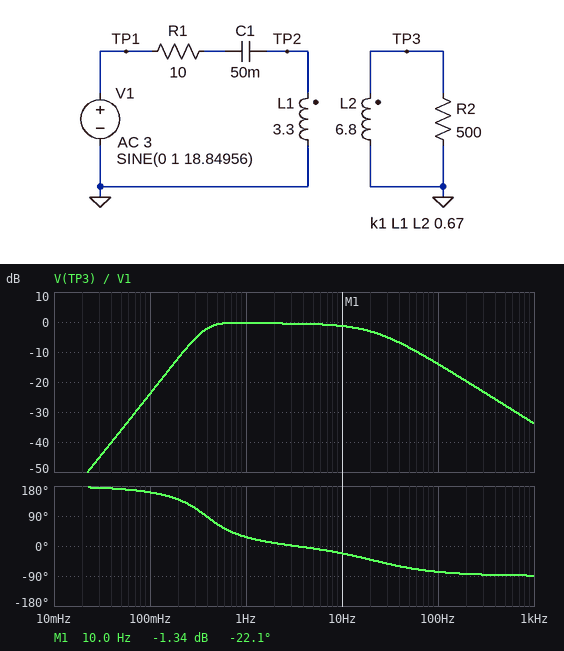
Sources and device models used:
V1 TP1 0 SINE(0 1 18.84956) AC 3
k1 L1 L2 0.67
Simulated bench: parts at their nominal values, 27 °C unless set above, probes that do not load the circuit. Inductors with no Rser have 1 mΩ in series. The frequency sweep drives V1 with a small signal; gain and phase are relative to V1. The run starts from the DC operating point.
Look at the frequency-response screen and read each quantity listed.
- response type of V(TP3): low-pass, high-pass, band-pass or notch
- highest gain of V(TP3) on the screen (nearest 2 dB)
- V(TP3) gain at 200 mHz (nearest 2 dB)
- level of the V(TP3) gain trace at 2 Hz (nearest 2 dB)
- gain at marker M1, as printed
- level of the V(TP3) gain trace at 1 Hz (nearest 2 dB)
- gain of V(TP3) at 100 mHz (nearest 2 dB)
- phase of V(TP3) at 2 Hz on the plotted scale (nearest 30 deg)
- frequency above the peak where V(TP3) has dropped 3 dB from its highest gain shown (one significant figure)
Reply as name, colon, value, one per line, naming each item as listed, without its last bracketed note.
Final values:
response type of V(TP3): low-pass, high-pass, band-pass or notch: band-pass
highest gain of V(TP3) on the screen: 0 dB
V(TP3) gain at 200 mHz: -12 dB
level of the V(TP3) gain trace at 2 Hz: 0 dB
gain at marker M1, as printed: -1.34 dB
level of the V(TP3) gain trace at 1 Hz: 0 dB
gain of V(TP3) at 100 mHz: -24 dB
phase of V(TP3) at 2 Hz on the plotted scale: 0 deg
frequency above the peak where V(TP3) has dropped 3 dB from its highest gain shown: 20 Hz
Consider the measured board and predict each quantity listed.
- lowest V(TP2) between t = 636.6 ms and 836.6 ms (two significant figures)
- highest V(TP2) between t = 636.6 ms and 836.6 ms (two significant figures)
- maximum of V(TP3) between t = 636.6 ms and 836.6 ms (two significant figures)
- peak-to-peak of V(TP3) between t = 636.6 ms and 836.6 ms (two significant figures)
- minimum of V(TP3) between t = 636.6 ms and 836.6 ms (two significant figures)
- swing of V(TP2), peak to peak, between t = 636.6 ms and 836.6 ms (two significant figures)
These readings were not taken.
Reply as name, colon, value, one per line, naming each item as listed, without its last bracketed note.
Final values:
lowest V(TP2) between t = 636.6 ms and 836.6 ms: -990 mV
highest V(TP2) between t = 636.6 ms and 836.6 ms: 990 mV
maximum of V(TP3) between t = 636.6 ms and 836.6 ms: 710 mV
peak-to-peak of V(TP3) between t = 636.6 ms and 836.6 ms: 1.4 V
minimum of V(TP3) between t = 636.6 ms and 836.6 ms: -720 mV
swing of V(TP2), peak to peak, between t = 636.6 ms and 836.6 ms: 2.0 V
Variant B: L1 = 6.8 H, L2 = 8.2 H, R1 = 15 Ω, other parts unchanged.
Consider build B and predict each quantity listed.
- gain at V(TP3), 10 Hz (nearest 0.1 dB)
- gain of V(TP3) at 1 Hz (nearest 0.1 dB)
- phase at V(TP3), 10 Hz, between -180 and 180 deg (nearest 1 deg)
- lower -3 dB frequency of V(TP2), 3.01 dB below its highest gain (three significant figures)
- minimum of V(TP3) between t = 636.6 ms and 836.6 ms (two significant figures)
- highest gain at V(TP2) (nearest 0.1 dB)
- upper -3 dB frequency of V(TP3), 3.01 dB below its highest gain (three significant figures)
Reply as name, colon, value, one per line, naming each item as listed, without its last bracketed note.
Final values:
gain at V(TP3), 10 Hz: -4.0 dB
gain of V(TP3) at 1 Hz: -2.7 dB
phase at V(TP3), 10 Hz, between -180 and 180 deg: -27 deg
lower -3 dB frequency of V(TP2), 3.01 dB below its highest gain: 252 mHz
minimum of V(TP3) between t = 636.6 ms and 836.6 ms: -500 mV
highest gain at V(TP2): 0 dB
upper -3 dB frequency of V(TP3), 3.01 dB below its highest gain: 17.4 Hz
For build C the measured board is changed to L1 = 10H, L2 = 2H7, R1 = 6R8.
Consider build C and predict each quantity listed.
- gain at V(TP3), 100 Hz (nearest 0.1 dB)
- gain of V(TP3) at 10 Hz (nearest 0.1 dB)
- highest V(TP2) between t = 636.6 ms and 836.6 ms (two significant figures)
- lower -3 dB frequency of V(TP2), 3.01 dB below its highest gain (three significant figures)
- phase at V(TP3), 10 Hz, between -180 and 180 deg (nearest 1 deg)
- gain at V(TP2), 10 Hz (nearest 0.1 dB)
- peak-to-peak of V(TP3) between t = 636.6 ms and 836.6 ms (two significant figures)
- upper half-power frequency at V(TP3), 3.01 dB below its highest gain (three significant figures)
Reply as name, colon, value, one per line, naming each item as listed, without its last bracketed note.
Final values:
gain at V(TP3), 100 Hz: -15.7 dB
gain of V(TP3) at 10 Hz: -9.3 dB
highest V(TP2) between t = 636.6 ms and 836.6 ms: 990 mV
lower -3 dB frequency of V(TP2), 3.01 dB below its highest gain: 193 mHz
phase at V(TP3), 10 Hz, between -180 and 180 deg: -10 deg
gain at V(TP2), 10 Hz: 0 dB
peak-to-peak of V(TP3) between t = 636.6 ms and 836.6 ms: 660 mV
upper half-power frequency at V(TP3), 3.01 dB below its highest gain: 350 mHz
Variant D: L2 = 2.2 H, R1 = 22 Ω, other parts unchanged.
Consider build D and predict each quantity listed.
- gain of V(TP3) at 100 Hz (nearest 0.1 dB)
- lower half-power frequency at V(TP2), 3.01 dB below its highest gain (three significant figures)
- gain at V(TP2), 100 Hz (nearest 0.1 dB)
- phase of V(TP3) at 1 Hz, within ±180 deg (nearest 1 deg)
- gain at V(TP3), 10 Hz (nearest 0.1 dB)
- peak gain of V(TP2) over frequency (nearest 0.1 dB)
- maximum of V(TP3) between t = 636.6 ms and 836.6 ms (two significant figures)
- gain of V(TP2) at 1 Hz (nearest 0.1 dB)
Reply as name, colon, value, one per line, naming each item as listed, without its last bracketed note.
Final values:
gain of V(TP3) at 100 Hz: -10.5 dB
lower half-power frequency at V(TP2), 3.01 dB below its highest gain: 932 mHz
gain at V(TP2), 100 Hz: 0 dB
phase of V(TP3) at 1 Hz, within ±180 deg: 50 deg
gain at V(TP3), 10 Hz: -5.5 dB
peak gain of V(TP2) over frequency: 0 dB
maximum of V(TP3) between t = 636.6 ms and 836.6 ms: 520 mV
gain of V(TP2) at 1 Hz: -2.7 dB
